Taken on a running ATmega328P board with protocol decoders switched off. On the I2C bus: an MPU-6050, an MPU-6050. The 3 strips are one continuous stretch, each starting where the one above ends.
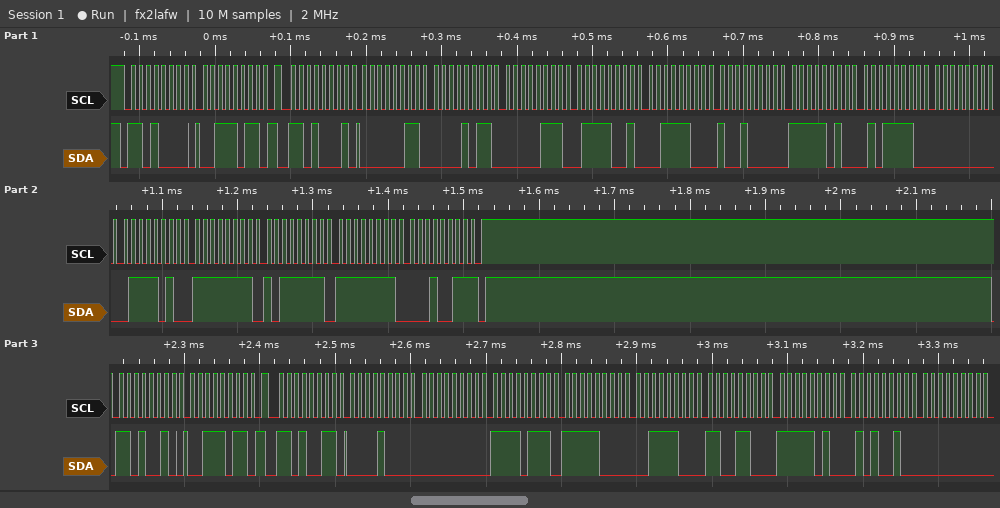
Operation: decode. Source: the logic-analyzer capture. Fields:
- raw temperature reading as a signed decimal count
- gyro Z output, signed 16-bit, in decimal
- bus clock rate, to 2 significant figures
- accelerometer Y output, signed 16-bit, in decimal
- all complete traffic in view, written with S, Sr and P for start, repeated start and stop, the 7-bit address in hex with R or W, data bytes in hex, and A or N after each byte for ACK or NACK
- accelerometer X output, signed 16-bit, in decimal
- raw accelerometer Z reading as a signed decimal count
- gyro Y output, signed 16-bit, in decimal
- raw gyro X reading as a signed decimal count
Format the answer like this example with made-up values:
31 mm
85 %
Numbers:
-1442
-237
100 kHz
1913
S 68W A 3B A Sr 68R A 03 A 0B A 07 A 79 A 3C A 90 A FA A 5E A 00 A 7A A FF A BF A FF A 13 N P S 69W A 3B A Sr 69R A 08 A 00 A F7 A F8 A 3C A CC A FA A 52 A 00 A
779
15504
-65
122
